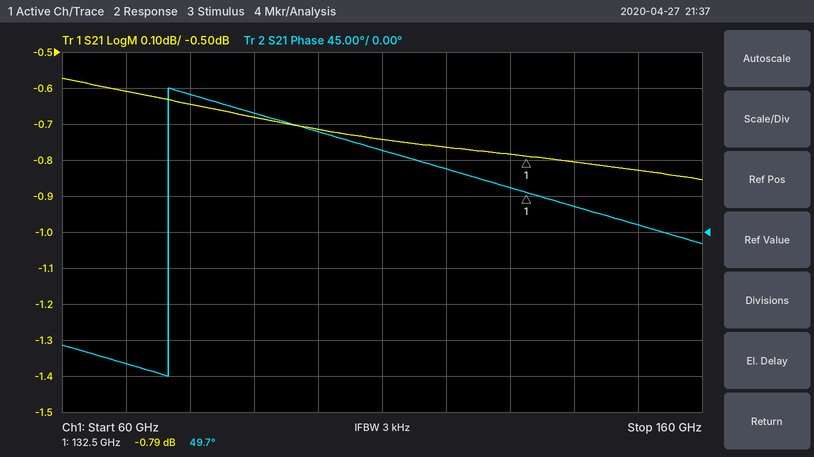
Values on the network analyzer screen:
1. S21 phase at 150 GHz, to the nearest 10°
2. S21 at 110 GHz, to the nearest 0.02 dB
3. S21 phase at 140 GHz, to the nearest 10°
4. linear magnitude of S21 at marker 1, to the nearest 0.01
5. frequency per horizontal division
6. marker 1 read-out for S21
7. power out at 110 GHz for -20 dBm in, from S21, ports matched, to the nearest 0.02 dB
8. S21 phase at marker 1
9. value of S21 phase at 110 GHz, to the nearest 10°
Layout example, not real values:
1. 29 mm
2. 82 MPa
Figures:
1. 10°
2. -0.74 dB
3. 30°
4. 0.91
5. 10 GHz
6. -0.79 dB
7. -20.74 dBm
8. 49.7°
9. 100°
